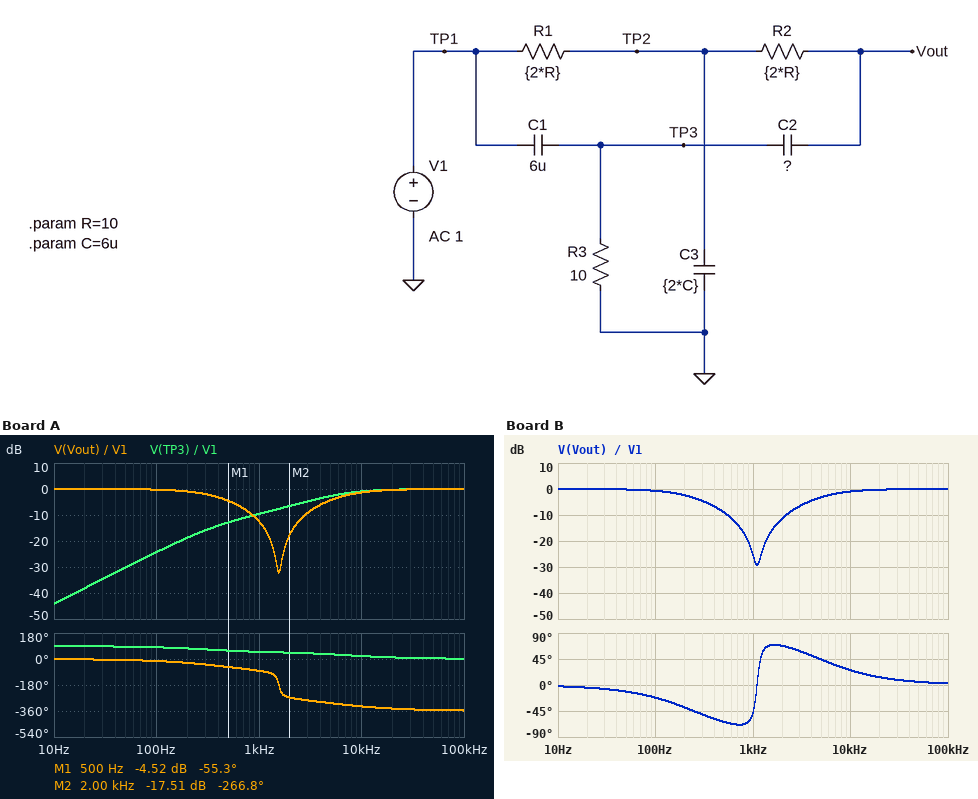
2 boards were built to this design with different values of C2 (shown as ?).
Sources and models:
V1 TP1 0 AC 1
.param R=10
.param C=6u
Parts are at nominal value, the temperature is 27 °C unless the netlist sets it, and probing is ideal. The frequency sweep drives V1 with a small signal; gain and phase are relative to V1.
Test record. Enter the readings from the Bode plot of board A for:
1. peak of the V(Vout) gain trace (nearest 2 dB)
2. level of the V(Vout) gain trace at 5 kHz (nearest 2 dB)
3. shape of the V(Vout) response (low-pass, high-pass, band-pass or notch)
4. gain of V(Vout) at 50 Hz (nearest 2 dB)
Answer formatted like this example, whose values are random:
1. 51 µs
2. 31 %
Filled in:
1. 0 dB
2. -4 dB
3. notch
4. 0 dB
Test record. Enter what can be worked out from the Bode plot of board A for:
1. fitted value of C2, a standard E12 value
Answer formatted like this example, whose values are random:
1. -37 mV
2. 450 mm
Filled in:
1. 3.9 µF
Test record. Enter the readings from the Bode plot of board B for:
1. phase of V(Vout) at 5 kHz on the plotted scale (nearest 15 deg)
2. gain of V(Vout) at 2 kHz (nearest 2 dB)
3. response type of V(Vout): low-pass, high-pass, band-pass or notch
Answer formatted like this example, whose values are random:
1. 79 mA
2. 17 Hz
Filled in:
1. 45 deg
2. -12 dB
3. notch
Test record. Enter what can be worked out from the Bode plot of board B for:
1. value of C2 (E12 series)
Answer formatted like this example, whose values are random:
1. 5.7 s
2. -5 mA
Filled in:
1. 10 µF
